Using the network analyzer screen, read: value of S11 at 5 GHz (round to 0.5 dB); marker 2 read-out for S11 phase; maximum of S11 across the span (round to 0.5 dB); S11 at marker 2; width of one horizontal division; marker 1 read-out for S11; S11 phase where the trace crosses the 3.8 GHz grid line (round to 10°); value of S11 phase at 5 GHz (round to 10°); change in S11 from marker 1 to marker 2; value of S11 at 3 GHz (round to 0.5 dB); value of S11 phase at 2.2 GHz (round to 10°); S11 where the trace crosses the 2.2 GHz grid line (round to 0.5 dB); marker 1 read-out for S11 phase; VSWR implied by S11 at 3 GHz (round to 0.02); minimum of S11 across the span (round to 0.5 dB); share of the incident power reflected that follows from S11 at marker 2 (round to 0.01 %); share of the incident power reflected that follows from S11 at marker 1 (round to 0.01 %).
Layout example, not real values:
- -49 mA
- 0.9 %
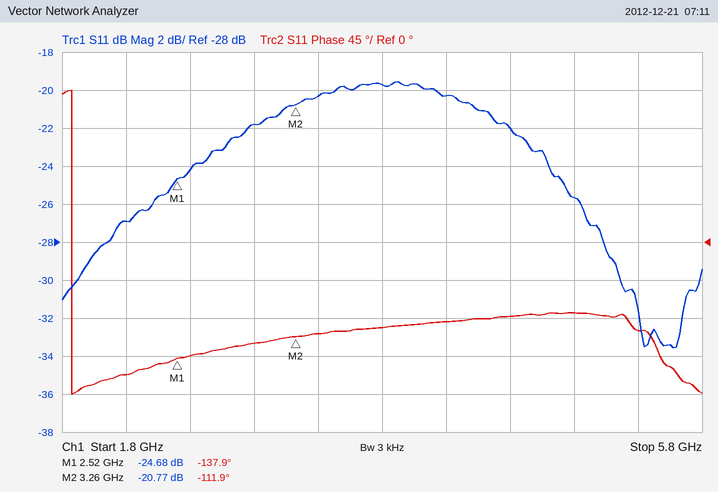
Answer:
- -25.5 dB
- -111.9°
- -19.5 dB
- -20.77 dB
- 400 MHz
- -24.68 dB
- -100°
- -80°
- 3.91 dB
- -22.0 dB
- -160°
- -27.0 dB
- -137.9°
- 1.18
- -33.5 dB
- 0.84 %
- 0.34 %
